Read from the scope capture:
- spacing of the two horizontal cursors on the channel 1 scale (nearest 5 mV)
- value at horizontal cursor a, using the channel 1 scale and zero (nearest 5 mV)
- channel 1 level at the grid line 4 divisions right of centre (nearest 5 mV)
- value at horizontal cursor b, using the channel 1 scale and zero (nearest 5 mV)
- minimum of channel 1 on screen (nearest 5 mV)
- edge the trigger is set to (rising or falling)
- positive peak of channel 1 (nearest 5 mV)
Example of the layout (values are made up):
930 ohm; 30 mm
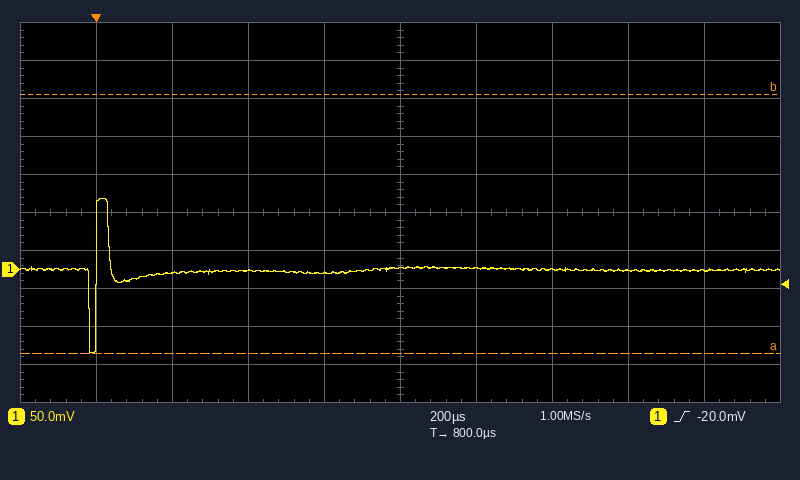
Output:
340 mV; -110 mV; 0 mV; 230 mV; -110 mV; rising; 95 mV
